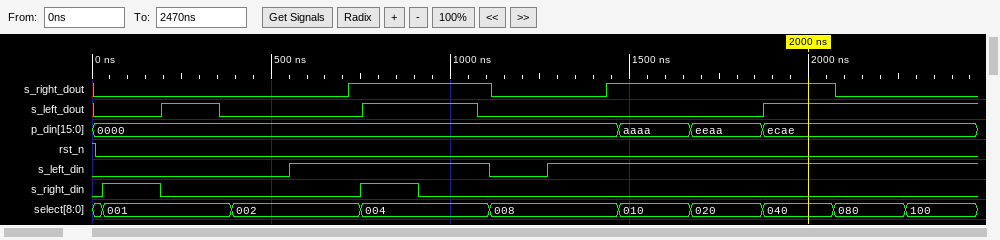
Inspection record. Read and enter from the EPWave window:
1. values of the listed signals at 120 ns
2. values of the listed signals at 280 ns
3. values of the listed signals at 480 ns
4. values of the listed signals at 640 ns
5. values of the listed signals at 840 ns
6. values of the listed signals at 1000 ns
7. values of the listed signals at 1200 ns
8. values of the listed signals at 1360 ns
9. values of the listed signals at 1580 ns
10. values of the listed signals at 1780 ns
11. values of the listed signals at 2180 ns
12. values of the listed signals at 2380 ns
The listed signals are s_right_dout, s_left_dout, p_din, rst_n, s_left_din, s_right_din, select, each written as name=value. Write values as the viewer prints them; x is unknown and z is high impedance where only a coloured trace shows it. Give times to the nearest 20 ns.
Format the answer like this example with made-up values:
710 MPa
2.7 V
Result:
s_right_dout=0, s_left_dout=0, p_din=0000, rst_n=0, s_left_din=0, s_right_din=1, select=001
s_right_dout=0, s_left_dout=1, p_din=0000, rst_n=0, s_left_din=0, s_right_din=0, select=001
s_right_dout=0, s_left_dout=0, p_din=0000, rst_n=0, s_left_din=0, s_right_din=0, select=002
s_right_dout=0, s_left_dout=0, p_din=0000, rst_n=0, s_left_din=1, s_right_din=0, select=002
s_right_dout=1, s_left_dout=1, p_din=0000, rst_n=0, s_left_din=1, s_right_din=1, select=004
s_right_dout=1, s_left_dout=1, p_din=0000, rst_n=0, s_left_din=1, s_right_din=0, select=004
s_right_dout=0, s_left_dout=0, p_din=0000, rst_n=0, s_left_din=0, s_right_din=0, select=008
s_right_dout=0, s_left_dout=0, p_din=0000, rst_n=0, s_left_din=1, s_right_din=0, select=008
s_right_dout=1, s_left_dout=0, p_din=aaaa, rst_n=0, s_left_din=1, s_right_din=0, select=010
s_right_dout=1, s_left_dout=0, p_din=eeaa, rst_n=0, s_left_din=1, s_right_din=0, select=020
s_right_dout=0, s_left_dout=1, p_din=ecae, rst_n=0, s_left_din=1, s_right_din=0, select=080
s_right_dout=0, s_left_dout=1, p_din=ecae, rst_n=0, s_left_din=1, s_right_din=0, select=100
